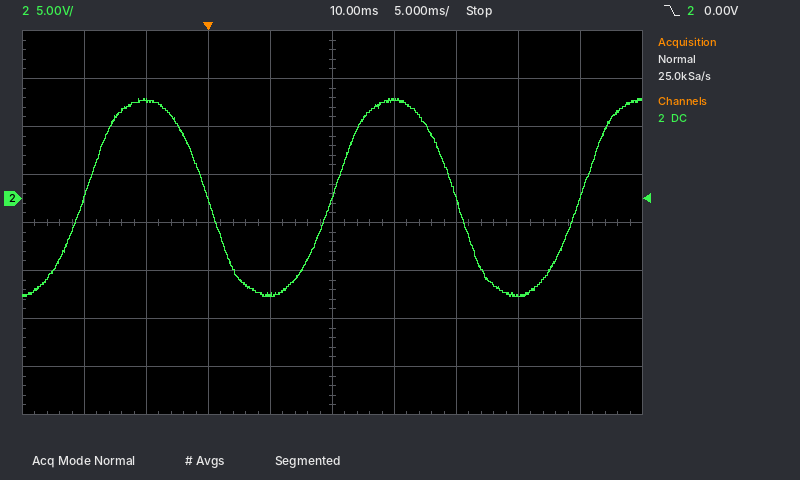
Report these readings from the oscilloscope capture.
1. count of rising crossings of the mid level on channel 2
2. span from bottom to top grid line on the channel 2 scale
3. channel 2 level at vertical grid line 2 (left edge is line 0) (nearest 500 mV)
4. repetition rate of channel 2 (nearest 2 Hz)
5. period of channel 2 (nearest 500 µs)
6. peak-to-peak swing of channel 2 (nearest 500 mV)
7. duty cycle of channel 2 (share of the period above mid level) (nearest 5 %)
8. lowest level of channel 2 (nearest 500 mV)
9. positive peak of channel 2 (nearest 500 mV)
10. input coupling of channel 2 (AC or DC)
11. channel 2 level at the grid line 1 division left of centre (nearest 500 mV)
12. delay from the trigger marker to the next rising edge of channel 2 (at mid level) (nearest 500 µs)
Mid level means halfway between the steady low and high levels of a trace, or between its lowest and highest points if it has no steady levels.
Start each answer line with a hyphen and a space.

- 3
- 40 V
- 10.0 V
- 50 Hz
- 20.0 ms
- 20.5 V
- 50 %
- -10.0 V
- 10.5 V
- DC
- -10.0 V
- 10.0 ms
